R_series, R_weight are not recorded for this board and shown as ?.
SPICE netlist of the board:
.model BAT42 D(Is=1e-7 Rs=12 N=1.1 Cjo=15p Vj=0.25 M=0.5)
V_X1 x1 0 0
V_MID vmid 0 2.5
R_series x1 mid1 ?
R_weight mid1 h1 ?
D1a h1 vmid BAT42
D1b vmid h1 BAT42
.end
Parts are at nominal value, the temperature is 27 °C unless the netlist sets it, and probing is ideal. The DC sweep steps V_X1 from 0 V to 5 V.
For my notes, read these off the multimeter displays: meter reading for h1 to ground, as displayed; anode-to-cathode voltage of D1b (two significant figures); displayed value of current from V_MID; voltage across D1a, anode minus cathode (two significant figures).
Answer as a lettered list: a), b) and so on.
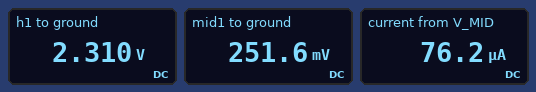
a) 2.310 V
b) 190 mV
c) 76.2 µA
d) -190 mV
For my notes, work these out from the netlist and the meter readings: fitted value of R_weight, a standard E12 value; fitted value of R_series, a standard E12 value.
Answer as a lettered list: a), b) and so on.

a) 27 kΩ
b) 3.3 kΩ
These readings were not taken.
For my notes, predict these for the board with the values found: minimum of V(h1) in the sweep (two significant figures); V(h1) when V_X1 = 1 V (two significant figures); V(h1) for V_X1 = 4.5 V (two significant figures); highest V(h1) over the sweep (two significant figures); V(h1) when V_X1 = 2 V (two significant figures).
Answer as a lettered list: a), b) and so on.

a) 2.3 V
b) 2.3 V
c) 2.7 V
d) 2.7 V
e) 2.4 V
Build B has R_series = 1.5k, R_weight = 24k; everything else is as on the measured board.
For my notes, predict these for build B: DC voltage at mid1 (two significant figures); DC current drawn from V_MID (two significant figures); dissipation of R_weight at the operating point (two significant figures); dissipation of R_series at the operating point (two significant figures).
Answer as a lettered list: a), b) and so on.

a) 140 mV
b) 90 µA
c) 200 µW
d) 12 µW
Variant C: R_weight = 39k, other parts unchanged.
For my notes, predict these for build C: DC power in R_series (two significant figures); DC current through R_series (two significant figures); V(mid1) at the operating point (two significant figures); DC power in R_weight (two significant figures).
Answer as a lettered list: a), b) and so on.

a) 9.9 µW
b) 55 µA
c) 180 mV
d) 120 µW
